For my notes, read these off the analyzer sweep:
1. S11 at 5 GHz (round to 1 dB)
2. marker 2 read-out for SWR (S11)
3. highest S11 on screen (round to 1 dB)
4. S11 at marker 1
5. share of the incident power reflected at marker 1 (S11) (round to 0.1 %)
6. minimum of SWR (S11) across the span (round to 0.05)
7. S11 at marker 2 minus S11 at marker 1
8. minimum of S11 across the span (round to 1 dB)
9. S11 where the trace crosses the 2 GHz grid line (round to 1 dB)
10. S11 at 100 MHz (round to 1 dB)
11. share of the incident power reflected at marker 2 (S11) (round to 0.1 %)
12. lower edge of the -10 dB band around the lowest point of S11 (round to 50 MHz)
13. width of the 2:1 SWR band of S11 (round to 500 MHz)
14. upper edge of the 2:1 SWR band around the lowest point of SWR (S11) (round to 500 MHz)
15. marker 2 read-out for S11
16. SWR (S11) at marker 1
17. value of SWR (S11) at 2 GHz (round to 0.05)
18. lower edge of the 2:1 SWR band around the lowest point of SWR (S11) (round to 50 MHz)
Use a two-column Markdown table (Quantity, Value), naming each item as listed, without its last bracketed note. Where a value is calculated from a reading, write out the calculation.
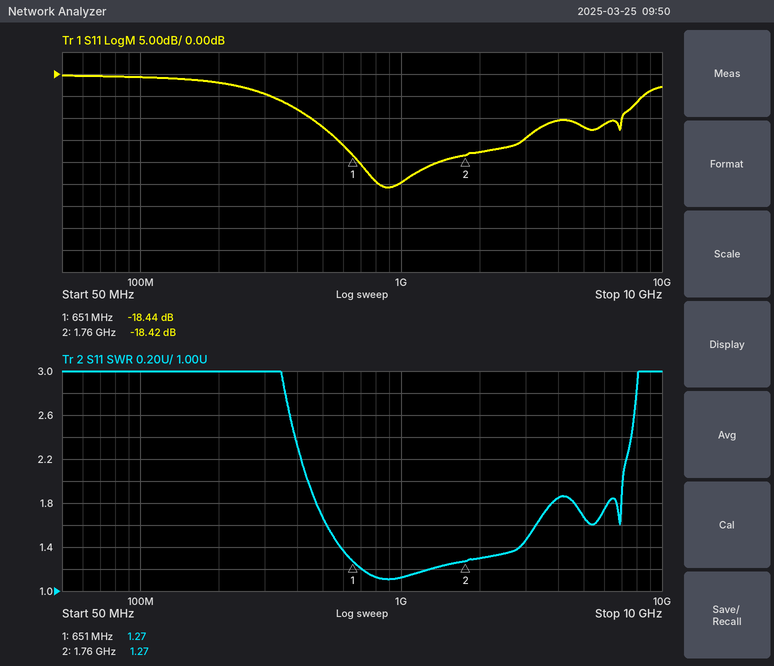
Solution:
| Quantity | Value |
|---|---|
| S11 at 5 GHz | -12 dB |
| marker 2 read-out for SWR | 1.27 |
| highest S11 on screen | 0 dB |
| S11 at marker 1 | -18.44 dB |
| share of the incident power reflected at marker 1 (S11) | 10^(-18.44/10) ≈ 1.4 % |
| minimum of SWR (S11) across the span | 1.10 |
| S11 at marker 2 minus S11 at marker 1 | -18.42 − (-18.44) = 0.02 dB |
| minimum of S11 across the span | -26 dB |
| S11 where the trace crosses the 2 GHz grid line | -18 dB |
| S11 at 100 MHz | -1 dB |
| share of the incident power reflected at marker 2 (S11) | 10^(-18.42/10) ≈ 1.4 % |
| lower edge of the -10 dB band around the lowest point of S11 | 450 MHz |
| width of the 2:1 SWR band of S11 | 7.0 GHz − 450 MHz = 6.55 GHz |
| upper edge of the 2:1 SWR band around the lowest point of SWR (S11) | 7.0 GHz |
| marker 2 read-out for S11 | -18.42 dB |
| SWR (S11) at marker 1 | 1.27 |
| value of SWR (S11) at 2 GHz | 1.30 |
| lower edge of the 2:1 SWR band around the lowest point of SWR (S11) | 450 MHz |
